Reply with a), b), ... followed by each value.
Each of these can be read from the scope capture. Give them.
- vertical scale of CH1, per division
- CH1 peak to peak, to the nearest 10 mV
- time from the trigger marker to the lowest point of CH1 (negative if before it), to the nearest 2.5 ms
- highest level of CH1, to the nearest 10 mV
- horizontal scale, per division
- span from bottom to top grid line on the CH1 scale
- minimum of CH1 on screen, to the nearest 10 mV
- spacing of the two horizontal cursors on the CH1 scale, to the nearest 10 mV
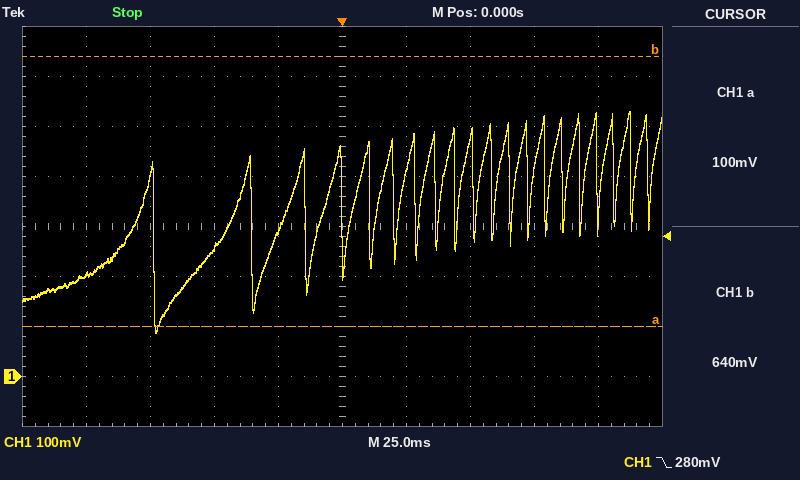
a) 100 mV
b) 440 mV
c) -72.5 ms
d) 530 mV
e) 25 ms
f) 800 mV
g) 90 mV
h) 540 mV
